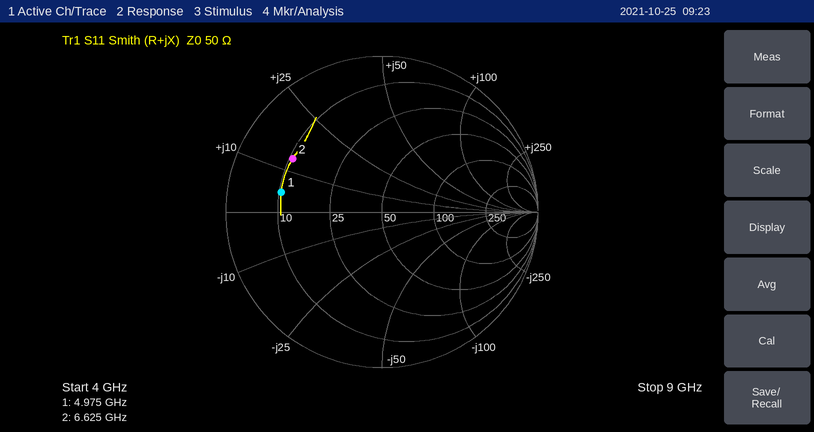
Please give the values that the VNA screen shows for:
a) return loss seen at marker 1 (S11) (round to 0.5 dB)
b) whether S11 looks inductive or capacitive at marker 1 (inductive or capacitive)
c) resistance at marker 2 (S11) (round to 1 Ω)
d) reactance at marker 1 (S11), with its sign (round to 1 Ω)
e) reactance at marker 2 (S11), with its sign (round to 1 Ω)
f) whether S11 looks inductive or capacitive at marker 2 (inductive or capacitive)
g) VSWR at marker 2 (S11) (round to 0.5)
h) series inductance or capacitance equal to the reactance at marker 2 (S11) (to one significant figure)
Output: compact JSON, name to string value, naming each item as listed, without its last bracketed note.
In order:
{"return loss seen at marker 1 (S11)": "3.5 dB", "whether S11 looks inductive or capacitive at marker 1": "inductive", "resistance at marker 2 (S11)": "11 Ω", "reactance at marker 1 (S11), with its sign": "+5 Ω", "reactance at marker 2 (S11), with its sign": "+13 Ω", "whether S11 looks inductive or capacitive at marker 2": "inductive", "VSWR at marker 2 (S11)": "5.0", "series inductance or capacitance equal to the reactance at marker 2 (S11)": "300 pH"}
